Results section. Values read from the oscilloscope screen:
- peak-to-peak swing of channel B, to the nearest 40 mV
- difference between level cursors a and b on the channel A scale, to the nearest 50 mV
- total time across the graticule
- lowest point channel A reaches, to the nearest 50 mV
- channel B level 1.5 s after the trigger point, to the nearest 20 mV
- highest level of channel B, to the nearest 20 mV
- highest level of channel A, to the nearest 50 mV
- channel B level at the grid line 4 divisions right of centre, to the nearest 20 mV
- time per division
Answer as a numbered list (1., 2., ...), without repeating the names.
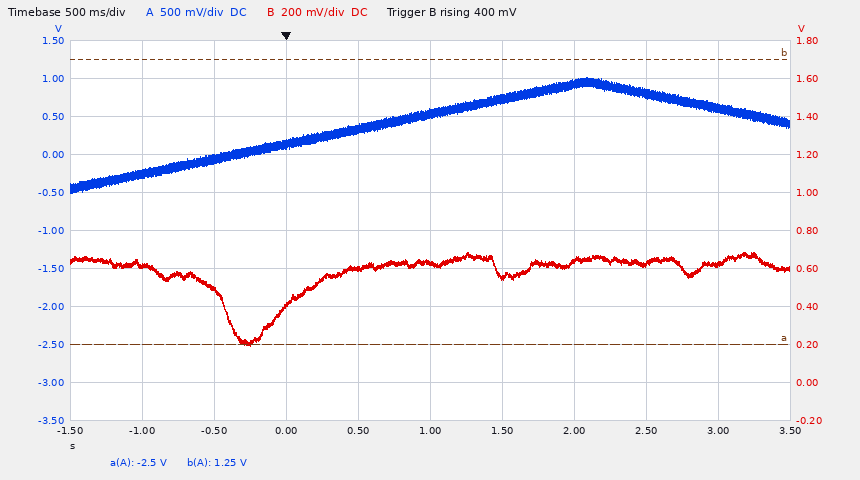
1. 480 mV
2. 3.75 V
3. 5 s
4. -500 mV
5. 560 mV
6. 680 mV
7. 1.00 V
8. 620 mV
9. 500 ms
